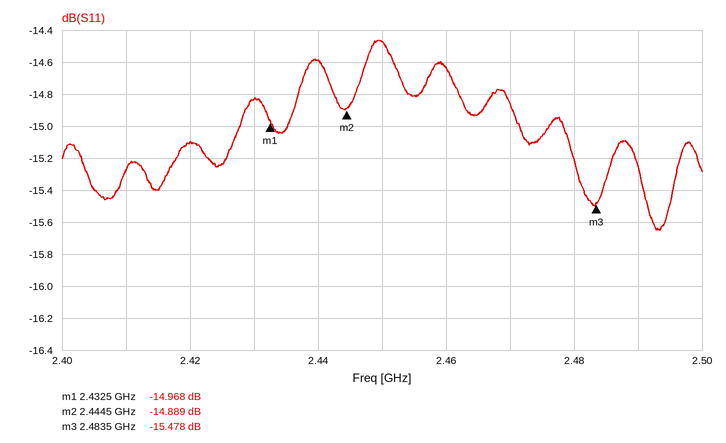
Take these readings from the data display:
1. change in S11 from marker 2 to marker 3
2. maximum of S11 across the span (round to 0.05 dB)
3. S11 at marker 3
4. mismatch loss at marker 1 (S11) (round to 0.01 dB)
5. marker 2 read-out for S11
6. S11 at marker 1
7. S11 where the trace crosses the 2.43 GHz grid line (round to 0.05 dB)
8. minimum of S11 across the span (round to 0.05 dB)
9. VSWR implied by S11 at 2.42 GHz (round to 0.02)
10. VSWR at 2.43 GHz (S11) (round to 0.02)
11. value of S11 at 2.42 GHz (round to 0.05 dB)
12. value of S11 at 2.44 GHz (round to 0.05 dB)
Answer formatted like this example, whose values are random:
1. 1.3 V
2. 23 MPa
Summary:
1. -0.589 dB
2. -14.45 dB
3. -15.478 dB
4. 0.14 dB
5. -14.889 dB
6. -14.968 dB
7. -14.85 dB
8. -15.65 dB
9. 1.42
10. 1.44
11. -15.10 dB
12. -14.60 dB
